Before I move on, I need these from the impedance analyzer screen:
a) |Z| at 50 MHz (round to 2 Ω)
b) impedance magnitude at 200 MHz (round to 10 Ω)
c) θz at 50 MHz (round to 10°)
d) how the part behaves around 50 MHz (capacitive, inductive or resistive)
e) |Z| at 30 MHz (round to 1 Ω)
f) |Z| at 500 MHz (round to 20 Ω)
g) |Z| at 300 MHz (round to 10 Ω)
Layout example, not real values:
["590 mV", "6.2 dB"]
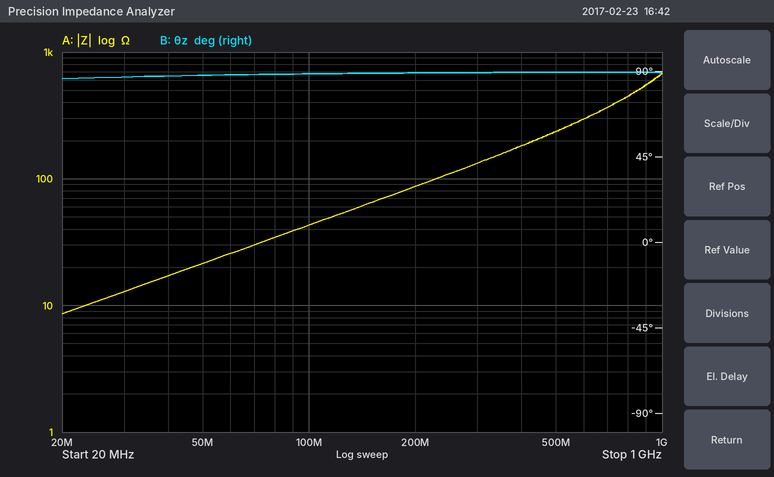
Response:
["22 Ω", "90 Ω", "90°", "inductive", "13 Ω", "240 Ω", "130 Ω"]
